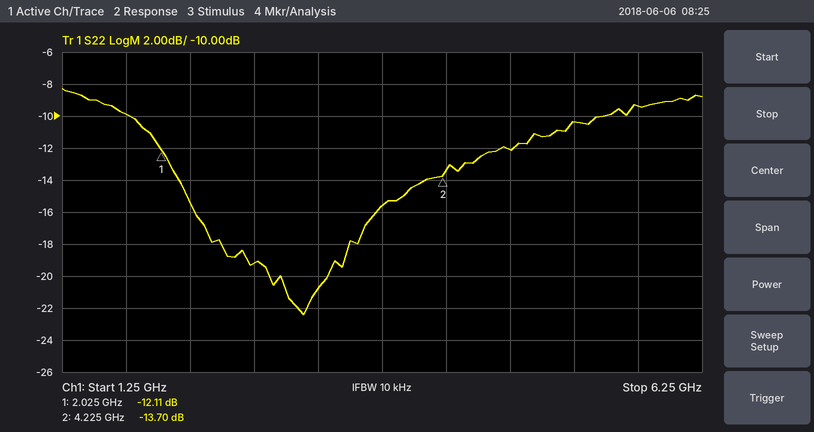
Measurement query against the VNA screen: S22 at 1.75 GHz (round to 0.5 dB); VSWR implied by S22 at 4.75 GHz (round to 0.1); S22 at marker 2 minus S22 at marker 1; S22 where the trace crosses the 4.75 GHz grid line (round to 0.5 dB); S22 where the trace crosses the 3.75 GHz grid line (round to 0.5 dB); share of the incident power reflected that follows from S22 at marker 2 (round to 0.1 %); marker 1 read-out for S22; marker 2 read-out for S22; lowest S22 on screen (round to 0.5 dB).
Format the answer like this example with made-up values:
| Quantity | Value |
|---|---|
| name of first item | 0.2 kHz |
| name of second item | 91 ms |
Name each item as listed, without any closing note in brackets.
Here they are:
| Quantity | Value |
|---|---|
| S22 at 1.75 GHz | -10.0 dB |
| VSWR implied by S22 at 4.75 GHz | 1.7 |
| S22 at marker 2 minus S22 at marker 1 | -1.59 dB |
| S22 where the trace crosses the 4.75 GHz grid line | -12.0 dB |
| S22 where the trace crosses the 3.75 GHz grid line | -15.5 dB |
| share of the incident power reflected that follows from S22 at marker 2 | 4.3 % |
| marker 1 read-out for S22 | -12.11 dB |
| marker 2 read-out for S22 | -13.70 dB |
| lowest S22 on screen | -22.5 dB |
